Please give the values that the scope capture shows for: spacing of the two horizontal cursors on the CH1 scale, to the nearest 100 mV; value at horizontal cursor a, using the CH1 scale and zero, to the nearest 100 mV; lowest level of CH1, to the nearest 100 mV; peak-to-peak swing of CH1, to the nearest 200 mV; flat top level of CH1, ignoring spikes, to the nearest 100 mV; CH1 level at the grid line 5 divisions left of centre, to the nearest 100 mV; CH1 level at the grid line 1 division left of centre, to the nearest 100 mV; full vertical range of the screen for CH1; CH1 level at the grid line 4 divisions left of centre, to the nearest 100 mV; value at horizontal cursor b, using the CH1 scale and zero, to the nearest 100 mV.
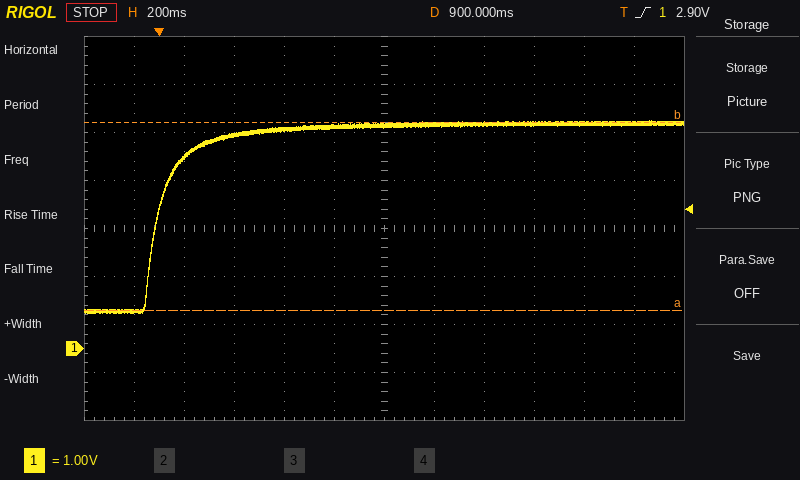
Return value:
3.9 V
800 mV
700 mV
4.0 V
4.7 V
800 mV
4.6 V
8 V
4.0 V
4.7 V
